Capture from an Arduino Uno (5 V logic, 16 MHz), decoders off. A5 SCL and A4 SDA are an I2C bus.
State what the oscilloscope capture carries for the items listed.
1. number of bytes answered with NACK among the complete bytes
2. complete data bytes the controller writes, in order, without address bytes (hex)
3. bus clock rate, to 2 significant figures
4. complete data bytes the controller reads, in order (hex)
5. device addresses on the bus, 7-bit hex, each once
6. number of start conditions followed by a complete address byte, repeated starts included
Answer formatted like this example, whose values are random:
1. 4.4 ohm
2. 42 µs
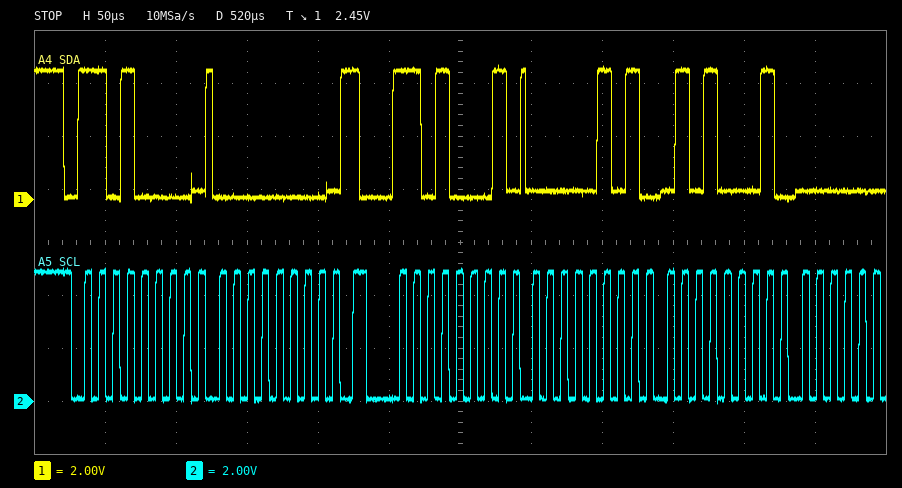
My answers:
1. 0
2. 00
3. 100 kHz
4. 05 51
5. 0x68
6. 2
